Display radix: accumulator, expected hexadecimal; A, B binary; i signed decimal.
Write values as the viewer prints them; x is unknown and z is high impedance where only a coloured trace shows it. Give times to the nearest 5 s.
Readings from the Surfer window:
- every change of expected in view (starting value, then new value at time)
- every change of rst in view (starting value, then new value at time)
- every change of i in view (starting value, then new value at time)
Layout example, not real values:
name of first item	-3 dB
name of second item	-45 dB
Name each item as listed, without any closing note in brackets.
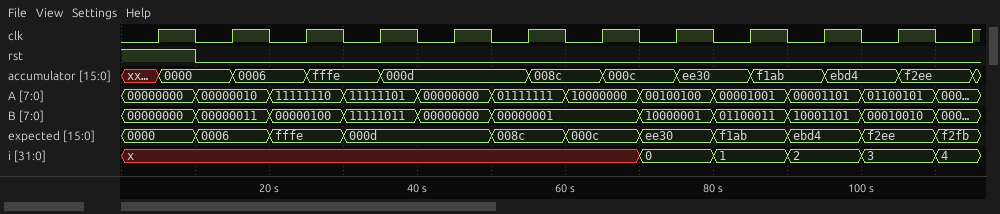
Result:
every change of expected in view	0000, 0006 at 10 s, fffe at 20 s, 000d at 30 s, 008c at 50 s, 000c at 60 s, ee30 at 70 s, f1ab at 80 s, ebd4 at 90 s, f2ee at 100 s, f2fb at 110 s
every change of rst in view	1, 0 at 10 s
every change of i in view	x, 0 at 70 s, 1 at 80 s, 2 at 90 s, 3 at 100 s, 4 at 110 s
